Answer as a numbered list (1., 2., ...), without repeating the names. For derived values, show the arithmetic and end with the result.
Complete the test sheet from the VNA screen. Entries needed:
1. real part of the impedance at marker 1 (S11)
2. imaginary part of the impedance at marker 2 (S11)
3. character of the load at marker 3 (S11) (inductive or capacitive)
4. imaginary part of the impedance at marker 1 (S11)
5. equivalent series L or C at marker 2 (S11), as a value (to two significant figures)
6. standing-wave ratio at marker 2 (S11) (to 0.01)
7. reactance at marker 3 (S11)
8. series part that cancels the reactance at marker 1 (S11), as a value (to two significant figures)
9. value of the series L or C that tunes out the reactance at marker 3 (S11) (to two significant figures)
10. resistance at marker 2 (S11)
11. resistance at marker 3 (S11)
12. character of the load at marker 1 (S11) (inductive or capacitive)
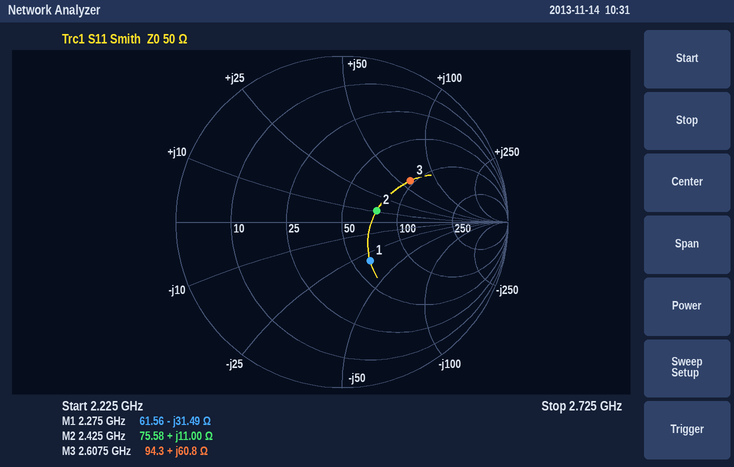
1. 61.56 Ω
2. +11.00 Ω
3. inductive
4. -31.49 Ω
5. L = 11 Ω/(2π × 2.425 GHz) ≈ 722 pH, so 720 pH to two significant figures
6. 1.57
7. +60.8 Ω
8. L = 31.49 Ω/(2π × 2.275 GHz) ≈ 2.2 nH
9. C = 1/(2π × 2.6075 GHz × 60.8 Ω) ≈ 1.0 pF
10. 75.58 Ω
11. 94.3 Ω
12. capacitive
